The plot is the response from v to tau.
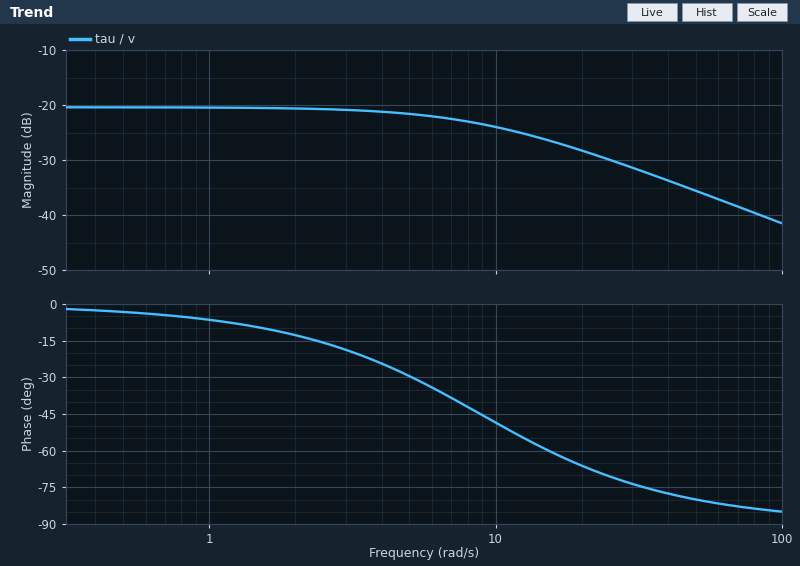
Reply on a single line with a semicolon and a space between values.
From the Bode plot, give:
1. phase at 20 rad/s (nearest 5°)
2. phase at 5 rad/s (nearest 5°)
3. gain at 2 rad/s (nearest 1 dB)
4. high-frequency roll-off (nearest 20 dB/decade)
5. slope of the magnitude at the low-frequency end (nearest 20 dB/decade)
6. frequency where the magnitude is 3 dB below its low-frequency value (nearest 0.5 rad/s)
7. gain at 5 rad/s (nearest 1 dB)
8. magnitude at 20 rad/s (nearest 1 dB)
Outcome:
-65°; -30°; -21 dB; -20 dB/decade; 0 dB/decade; 9.0 rad/s; -22 dB; -28 dB
